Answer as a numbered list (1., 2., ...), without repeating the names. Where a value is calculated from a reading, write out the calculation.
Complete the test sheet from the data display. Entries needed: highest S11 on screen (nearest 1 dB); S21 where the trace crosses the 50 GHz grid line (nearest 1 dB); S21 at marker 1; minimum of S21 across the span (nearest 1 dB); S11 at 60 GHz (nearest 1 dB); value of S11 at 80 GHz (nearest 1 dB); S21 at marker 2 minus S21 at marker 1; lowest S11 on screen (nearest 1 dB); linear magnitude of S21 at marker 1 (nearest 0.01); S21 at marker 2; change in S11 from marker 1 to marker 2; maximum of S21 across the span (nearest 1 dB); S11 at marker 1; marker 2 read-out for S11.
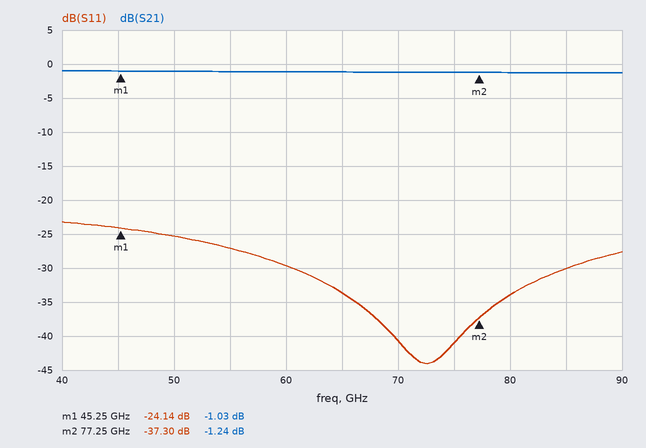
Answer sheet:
1. -23 dB
2. -1 dB
3. -1.03 dB
4. -1 dB
5. -30 dB
6. -34 dB
7. -1.24 − (-1.03) = -0.21 dB
8. -44 dB
9. 10^(-1.03/20) ≈ 0.89
10. -1.24 dB
11. -37.3 − (-24.14) = -13.16 dB
12. -1 dB
13. -24.14 dB
14. -37.30 dB
